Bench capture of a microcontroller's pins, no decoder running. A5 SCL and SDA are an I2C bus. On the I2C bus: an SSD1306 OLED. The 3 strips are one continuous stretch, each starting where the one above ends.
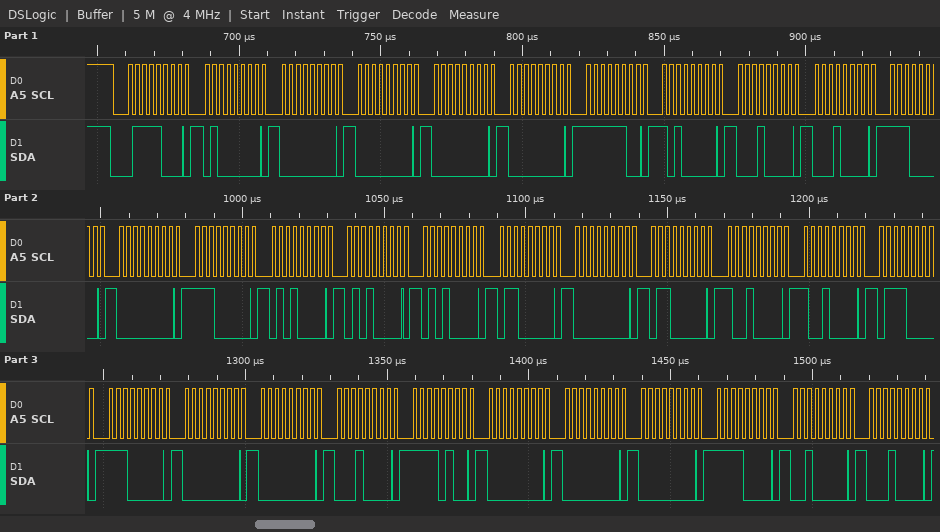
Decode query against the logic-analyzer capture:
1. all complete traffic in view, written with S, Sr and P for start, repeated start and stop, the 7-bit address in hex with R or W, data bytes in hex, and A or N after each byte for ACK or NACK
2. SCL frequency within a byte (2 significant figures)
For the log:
S 3CW A 40 A 00 A 00 A 00 A 00 A FC A A0 A 10 A 10 A E0 A 00 A E0 A 50 A 50 A 50 A 60 A 00 A 60 A 90 A 90 A 70 A E0 A 00 A 00 A 10 A F4 A 00 A 00 A 00 A F0 A 20 A 10 A
400 kHz
